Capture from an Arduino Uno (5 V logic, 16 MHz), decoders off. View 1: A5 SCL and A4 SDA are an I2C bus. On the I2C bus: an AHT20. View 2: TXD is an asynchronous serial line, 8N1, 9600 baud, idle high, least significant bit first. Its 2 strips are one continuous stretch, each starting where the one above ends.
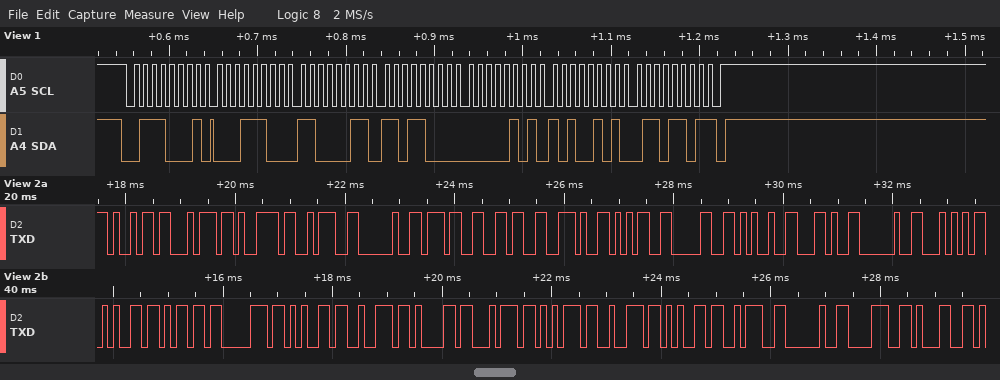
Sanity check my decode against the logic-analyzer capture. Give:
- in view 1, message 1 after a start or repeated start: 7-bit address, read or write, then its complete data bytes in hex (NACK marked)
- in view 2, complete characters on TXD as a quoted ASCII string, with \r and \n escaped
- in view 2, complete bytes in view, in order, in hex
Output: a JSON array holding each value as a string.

["0x38 read: 1C C3 D8 05 A5 6D NACK", "\"ity: 76.50%, Temperature: 81\"", "69 74 79 3A 20 37 36 2E 35 30 25 2C 20 54 65 6D 70 65 72 61 74 75 72 65 3A 20 38 31"]
